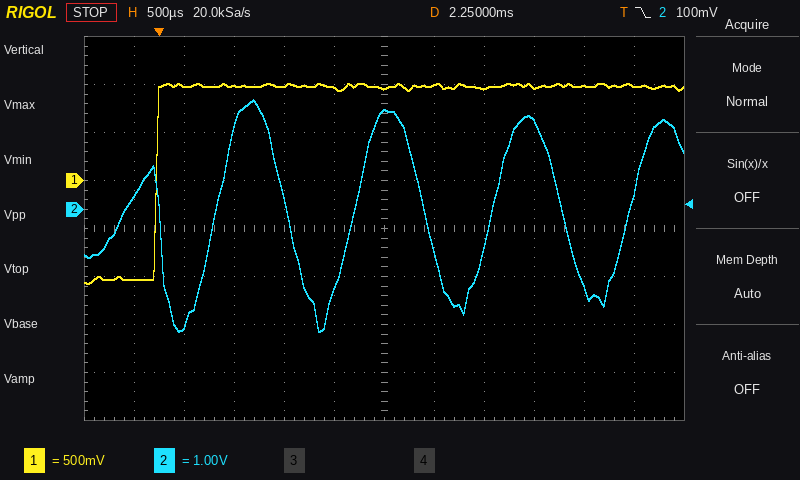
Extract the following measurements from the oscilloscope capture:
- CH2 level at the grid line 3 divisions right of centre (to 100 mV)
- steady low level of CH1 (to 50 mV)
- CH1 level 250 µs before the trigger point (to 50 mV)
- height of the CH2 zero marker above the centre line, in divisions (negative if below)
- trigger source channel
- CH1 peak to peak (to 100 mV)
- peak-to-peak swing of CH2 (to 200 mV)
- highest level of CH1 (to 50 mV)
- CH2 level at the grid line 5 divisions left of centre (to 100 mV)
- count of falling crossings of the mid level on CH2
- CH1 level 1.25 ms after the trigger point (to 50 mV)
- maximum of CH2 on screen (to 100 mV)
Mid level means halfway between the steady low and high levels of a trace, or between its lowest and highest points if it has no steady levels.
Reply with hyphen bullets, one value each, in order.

- 1.8 V
- -1.05 V
- -1.05 V
- +0.4 div
- CH2
- 2.10 V
- 4.8 V
- 1.00 V
- 300 mV
- 4
- 1.00 V
- 2.3 V
